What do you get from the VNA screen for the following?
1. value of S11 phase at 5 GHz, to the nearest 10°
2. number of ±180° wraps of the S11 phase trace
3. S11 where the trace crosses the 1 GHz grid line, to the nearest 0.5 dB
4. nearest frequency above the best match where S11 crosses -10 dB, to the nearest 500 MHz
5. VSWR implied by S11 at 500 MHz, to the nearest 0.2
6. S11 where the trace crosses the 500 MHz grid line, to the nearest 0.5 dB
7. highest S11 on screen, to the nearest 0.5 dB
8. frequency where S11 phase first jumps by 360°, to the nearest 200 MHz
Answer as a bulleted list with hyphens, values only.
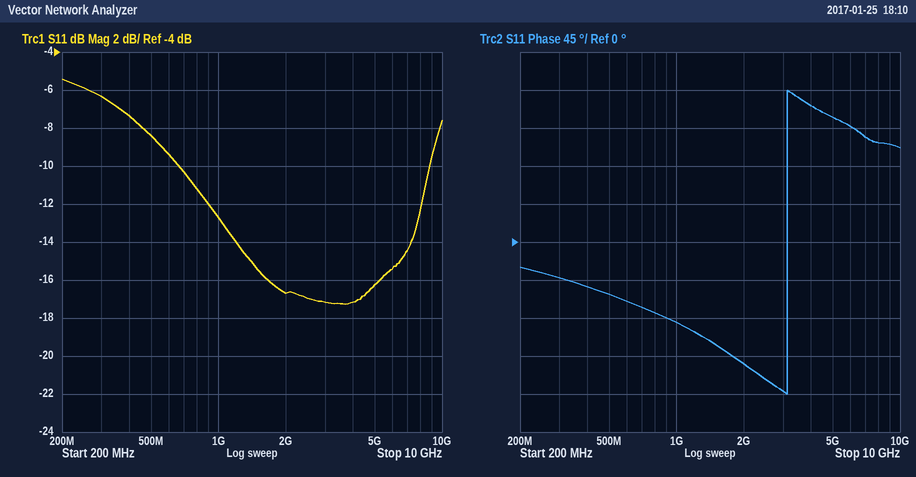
- 150°
- 1
- -12.5 dB
- 9.0 GHz
- 2.2
- -8.5 dB
- -5.5 dB
- 3.2 GHz
